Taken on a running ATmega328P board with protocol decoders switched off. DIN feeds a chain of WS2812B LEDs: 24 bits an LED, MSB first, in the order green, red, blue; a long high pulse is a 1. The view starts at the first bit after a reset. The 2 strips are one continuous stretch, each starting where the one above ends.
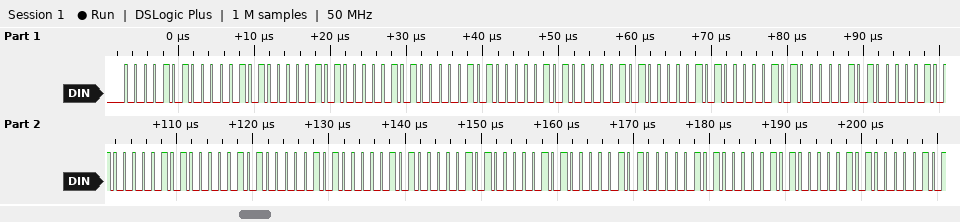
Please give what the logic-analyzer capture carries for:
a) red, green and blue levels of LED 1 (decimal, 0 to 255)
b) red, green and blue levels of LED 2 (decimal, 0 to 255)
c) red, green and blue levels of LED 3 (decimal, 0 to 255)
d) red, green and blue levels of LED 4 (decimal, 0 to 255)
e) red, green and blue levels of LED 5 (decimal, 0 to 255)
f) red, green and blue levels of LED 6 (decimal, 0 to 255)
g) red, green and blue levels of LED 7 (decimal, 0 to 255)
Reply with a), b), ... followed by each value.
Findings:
a) 10, 10, 10
b) 10, 10, 10
c) 10, 10, 10
d) 10, 10, 10
e) 10, 10, 10
f) 10, 10, 10
g) 10, 10, 10
